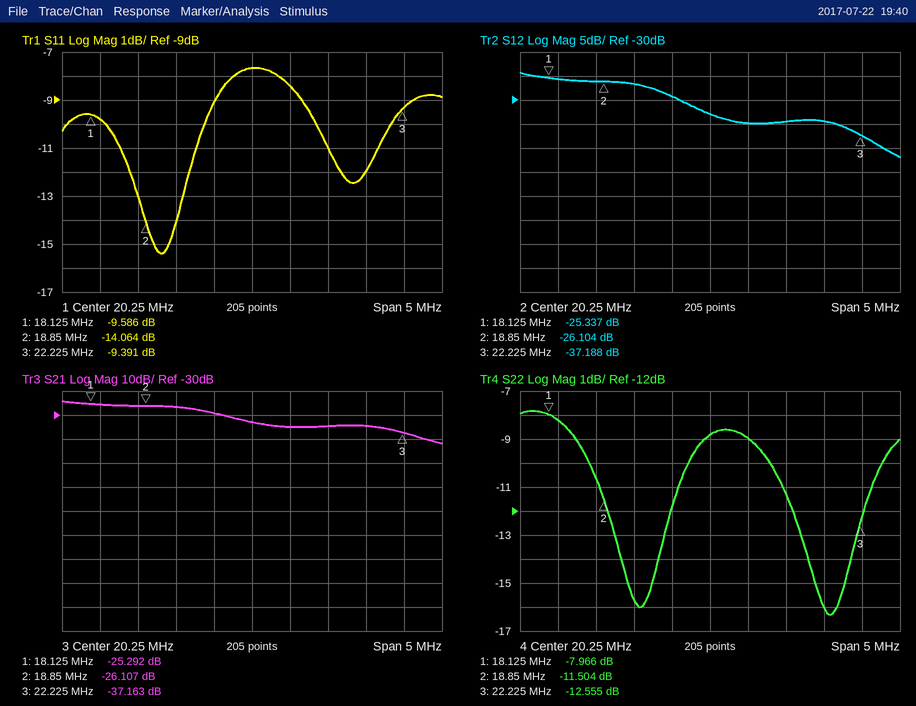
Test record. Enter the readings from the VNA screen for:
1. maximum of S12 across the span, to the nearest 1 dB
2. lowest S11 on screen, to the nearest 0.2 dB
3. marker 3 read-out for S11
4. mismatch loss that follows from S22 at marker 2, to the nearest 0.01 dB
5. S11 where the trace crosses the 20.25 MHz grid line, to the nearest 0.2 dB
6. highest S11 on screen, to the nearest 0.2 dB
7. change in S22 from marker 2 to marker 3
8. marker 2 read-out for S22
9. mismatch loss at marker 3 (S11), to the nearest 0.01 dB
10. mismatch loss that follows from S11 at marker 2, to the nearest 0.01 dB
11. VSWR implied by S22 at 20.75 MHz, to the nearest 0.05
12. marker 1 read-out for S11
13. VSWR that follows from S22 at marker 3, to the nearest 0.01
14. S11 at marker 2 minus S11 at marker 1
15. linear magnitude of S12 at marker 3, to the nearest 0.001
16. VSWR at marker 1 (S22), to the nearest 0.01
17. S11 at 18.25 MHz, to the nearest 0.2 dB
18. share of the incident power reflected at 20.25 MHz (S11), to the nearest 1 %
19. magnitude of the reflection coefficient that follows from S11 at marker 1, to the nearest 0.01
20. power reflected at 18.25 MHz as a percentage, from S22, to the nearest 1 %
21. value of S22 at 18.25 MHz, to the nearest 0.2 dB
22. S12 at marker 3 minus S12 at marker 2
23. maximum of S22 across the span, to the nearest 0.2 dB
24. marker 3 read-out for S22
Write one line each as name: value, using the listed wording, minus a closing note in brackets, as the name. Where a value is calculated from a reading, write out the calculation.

maximum of S12 across the span, to the nearest 1 dB: -24 dB
lowest S11 on screen, to the nearest 0.2 dB: -15.4 dB
marker 3 read-out for S11: -9.391 dB
mismatch loss that follows from S22 at marker 2, to the nearest 0.01 dB: −10 log10(1 − 10^(-11.504/10)) ≈ 0.32 dB
S11 where the trace crosses the 20.25 MHz grid line, to the nearest 0.2 dB: -7.6 dB
highest S11 on screen, to the nearest 0.2 dB: -7.6 dB
change in S22 from marker 2 to marker 3: -12.555 − (-11.504) = -1.051 dB
marker 2 read-out for S22: -11.504 dB
mismatch loss at marker 3 (S11), to the nearest 0.01 dB: −10 log10(1 − 10^(-9.391/10)) ≈ 0.53 dB
mismatch loss that follows from S11 at marker 2, to the nearest 0.01 dB: −10 log10(1 − 10^(-14.064/10)) ≈ 0.17 dB
VSWR implied by S22 at 20.75 MHz, to the nearest 0.05: |Γ| = 10^(-9/20) = 0.3548; VSWR = (1 + 0.3548)/(1 − 0.3548) ≈ 2.10
marker 1 read-out for S11: -9.586 dB
VSWR that follows from S22 at marker 3, to the nearest 0.01: (1 + 0.2356)/(1 − 0.2356) ≈ 1.62
S11 at marker 2 minus S11 at marker 1: -14.064 − (-9.586) = -4.478 dB
linear magnitude of S12 at marker 3, to the nearest 0.001: 10^(-37.188/20) ≈ 0.014
VSWR at marker 1 (S22), to the nearest 0.01: (1 + 0.3997)/(1 − 0.3997) ≈ 2.33
S11 at 18.25 MHz, to the nearest 0.2 dB: -9.8 dB
share of the incident power reflected at 20.25 MHz (S11), to the nearest 1 %: 10^(-7.6/10) ≈ 17 %
magnitude of the reflection coefficient that follows from S11 at marker 1, to the nearest 0.01: 10^(-9.586/20) ≈ 0.33
power reflected at 18.25 MHz as a percentage, from S22, to the nearest 1 %: 10^(-8.2/10) ≈ 15 %
value of S22 at 18.25 MHz, to the nearest 0.2 dB: -8.2 dB
S12 at marker 3 minus S12 at marker 2: -37.188 − (-26.104) = -11.084 dB
maximum of S22 across the span, to the nearest 0.2 dB: -7.8 dB
marker 3 read-out for S22: -12.555 dB
